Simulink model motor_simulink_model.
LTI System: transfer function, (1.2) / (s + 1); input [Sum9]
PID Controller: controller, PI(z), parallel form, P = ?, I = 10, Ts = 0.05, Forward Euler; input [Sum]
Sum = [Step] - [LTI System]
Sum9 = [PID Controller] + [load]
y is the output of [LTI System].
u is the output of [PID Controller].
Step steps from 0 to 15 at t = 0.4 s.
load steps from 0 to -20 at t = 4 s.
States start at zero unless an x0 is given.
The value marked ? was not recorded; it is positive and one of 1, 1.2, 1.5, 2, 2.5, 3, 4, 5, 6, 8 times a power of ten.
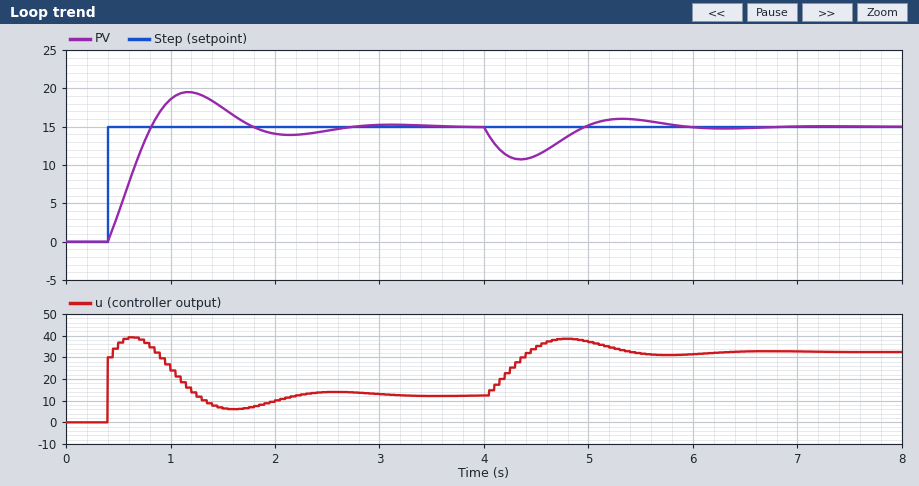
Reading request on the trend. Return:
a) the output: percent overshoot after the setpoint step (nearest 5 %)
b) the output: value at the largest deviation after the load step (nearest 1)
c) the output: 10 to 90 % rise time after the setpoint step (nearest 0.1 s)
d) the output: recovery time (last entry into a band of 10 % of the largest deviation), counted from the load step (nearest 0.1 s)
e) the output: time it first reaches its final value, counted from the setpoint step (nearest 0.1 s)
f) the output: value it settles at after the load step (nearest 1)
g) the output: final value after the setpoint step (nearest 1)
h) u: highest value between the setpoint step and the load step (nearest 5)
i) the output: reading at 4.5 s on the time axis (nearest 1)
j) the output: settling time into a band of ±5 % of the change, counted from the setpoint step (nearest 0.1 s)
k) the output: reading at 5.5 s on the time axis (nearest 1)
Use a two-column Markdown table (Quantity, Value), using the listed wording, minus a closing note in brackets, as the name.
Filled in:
| Quantity | Value |
|---|---|
| the output: percent overshoot after the setpoint step | 30 % |
| the output: value at the largest deviation after the load step | 11 |
| the output: 10 to 90 % rise time after the setpoint step | 0.3 s |
| the output: recovery time (last entry into a band of 10 % of the largest deviation), counted from the load step | 1.7 s |
| the output: time it first reaches its final value, counted from the setpoint step | 0.4 s |
| the output: value it settles at after the load step | 15 |
| the output: final value after the setpoint step | 15 |
| u: highest value between the setpoint step and the load step | 40 |
| the output: reading at 4.5 s on the time axis | 11 |
| the output: settling time into a band of ±5 % of the change, counted from the setpoint step | 2.0 s |
| the output: reading at 5.5 s on the time axis | 16 |
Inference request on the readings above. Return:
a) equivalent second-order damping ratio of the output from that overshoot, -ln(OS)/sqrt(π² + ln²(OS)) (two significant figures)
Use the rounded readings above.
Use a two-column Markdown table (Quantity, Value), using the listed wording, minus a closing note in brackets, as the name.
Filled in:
| Quantity | Value |
|---|---|
| equivalent second-order damping ratio of the output from that overshoot, -ln(OS)/sqrt(π² + ln²(OS)) | 0.36 |
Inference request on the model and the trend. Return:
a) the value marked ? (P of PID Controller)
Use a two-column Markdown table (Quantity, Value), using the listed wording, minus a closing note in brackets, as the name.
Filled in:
| Quantity | Value |
|---|---|
| the value marked ? | 2 |
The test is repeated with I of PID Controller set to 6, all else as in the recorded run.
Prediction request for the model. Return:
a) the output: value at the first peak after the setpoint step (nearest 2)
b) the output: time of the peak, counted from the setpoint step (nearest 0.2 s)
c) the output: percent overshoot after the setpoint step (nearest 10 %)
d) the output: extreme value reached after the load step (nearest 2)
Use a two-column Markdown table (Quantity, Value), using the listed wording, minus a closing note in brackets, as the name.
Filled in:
| Quantity | Value |
|---|---|
| the output: value at the first peak after the setpoint step | 18 |
| the output: time of the peak, counted from the setpoint step | 1.0 s |
| the output: percent overshoot after the setpoint step | 20 % |
| the output: extreme value reached after the load step | 10 |
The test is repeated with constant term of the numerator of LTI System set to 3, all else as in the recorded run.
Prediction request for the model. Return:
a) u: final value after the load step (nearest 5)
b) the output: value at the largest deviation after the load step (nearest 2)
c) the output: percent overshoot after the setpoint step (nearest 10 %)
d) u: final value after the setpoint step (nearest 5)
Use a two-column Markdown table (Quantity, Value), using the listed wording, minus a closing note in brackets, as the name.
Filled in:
| Quantity | Value |
|---|---|
| u: final value after the load step | 25 |
| the output: value at the largest deviation after the load step | 8 |
| the output: percent overshoot after the setpoint step | 30 % |
| u: final value after the setpoint step | 5 |
